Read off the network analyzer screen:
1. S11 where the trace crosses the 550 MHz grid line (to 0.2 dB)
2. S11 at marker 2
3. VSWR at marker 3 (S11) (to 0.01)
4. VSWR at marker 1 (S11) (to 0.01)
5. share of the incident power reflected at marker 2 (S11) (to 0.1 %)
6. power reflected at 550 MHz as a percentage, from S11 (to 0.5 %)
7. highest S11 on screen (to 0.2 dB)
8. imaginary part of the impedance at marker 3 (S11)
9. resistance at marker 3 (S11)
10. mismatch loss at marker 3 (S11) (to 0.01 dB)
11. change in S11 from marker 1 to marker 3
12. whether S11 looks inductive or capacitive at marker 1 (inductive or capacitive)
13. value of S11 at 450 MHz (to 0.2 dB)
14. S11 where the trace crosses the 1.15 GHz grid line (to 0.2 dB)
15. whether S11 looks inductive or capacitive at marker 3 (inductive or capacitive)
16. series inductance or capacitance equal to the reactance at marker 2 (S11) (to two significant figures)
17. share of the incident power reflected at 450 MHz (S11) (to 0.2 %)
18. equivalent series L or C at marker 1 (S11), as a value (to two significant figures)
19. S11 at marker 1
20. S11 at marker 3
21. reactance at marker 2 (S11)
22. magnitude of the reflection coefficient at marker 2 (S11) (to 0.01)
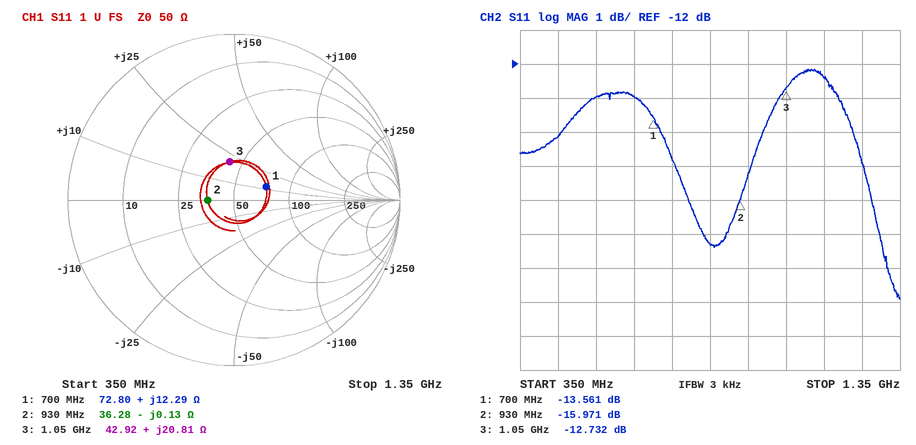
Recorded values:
-13.0 dB
-15.971 dB
1.60
1.53
2.5 %
5.0 %
-12.2 dB
+20.81 Ω
42.92 Ω
0.24 dB
0.829 dB
inductive
-14.2 dB
-12.4 dB
inductive
1.3 nF
3.8 %
2.8 nH
-13.561 dB
-12.732 dB
-0.13 Ω
0.16
